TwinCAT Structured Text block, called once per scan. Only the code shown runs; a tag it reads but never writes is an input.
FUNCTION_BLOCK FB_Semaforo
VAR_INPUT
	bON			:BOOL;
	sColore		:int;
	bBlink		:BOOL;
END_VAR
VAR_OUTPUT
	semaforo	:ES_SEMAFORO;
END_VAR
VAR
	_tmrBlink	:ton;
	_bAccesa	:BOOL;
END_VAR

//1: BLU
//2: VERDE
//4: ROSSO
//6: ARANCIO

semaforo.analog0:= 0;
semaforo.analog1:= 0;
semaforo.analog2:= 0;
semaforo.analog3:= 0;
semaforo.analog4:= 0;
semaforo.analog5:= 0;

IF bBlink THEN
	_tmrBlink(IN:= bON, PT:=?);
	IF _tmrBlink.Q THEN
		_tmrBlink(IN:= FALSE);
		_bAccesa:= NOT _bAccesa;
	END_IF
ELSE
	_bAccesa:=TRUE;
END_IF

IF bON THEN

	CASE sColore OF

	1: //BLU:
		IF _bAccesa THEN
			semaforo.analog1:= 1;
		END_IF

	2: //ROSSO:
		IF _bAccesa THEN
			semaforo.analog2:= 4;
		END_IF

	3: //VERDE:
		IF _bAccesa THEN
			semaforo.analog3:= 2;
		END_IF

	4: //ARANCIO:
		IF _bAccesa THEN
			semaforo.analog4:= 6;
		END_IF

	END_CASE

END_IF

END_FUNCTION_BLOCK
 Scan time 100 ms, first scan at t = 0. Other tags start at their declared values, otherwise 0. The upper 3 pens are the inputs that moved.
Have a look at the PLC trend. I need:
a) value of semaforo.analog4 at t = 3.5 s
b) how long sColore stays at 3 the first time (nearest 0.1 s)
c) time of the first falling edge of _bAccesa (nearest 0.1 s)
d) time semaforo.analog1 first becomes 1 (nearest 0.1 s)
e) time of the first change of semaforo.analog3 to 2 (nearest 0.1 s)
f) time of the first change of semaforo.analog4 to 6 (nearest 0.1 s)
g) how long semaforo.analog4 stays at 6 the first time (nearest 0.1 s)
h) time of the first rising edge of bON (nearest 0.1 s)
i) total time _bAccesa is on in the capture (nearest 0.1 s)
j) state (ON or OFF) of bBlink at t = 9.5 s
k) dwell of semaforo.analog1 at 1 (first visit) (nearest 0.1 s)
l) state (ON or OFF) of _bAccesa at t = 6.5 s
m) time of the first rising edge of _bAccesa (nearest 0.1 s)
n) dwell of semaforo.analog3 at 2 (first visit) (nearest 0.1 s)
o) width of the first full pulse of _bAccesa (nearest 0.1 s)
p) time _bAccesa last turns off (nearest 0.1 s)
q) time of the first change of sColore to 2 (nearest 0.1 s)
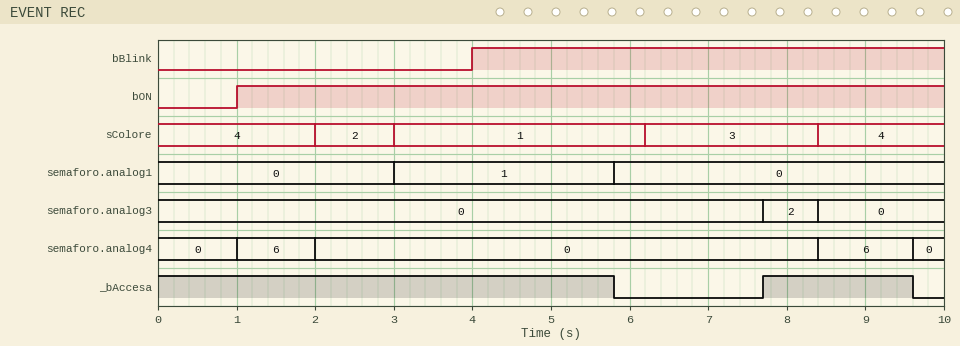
0
2.2 s
5.8 s
3.0 s
7.7 s
1.0 s
1.0 s
1.0 s
7.7 s
ON
2.8 s
OFF
7.7 s
0.7 s
1.9 s
9.6 s
2.0 s
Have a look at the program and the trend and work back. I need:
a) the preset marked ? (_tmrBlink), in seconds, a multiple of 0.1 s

1.8 s
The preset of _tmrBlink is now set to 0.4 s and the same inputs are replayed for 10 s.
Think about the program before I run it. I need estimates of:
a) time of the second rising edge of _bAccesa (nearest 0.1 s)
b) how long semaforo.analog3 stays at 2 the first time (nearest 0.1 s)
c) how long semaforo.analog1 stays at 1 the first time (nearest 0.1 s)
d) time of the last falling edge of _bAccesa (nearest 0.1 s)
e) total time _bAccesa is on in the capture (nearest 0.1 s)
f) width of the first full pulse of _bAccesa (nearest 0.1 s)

5.9 s
0.2 s
1.4 s
9.4 s
7.0 s
0.5 s
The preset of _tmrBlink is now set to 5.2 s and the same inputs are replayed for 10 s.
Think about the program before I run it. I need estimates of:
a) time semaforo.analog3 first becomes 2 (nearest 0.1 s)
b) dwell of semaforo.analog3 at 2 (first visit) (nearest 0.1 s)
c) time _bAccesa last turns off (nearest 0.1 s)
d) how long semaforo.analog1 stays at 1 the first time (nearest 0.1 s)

6.2 s
2.2 s
9.2 s
3.2 s
